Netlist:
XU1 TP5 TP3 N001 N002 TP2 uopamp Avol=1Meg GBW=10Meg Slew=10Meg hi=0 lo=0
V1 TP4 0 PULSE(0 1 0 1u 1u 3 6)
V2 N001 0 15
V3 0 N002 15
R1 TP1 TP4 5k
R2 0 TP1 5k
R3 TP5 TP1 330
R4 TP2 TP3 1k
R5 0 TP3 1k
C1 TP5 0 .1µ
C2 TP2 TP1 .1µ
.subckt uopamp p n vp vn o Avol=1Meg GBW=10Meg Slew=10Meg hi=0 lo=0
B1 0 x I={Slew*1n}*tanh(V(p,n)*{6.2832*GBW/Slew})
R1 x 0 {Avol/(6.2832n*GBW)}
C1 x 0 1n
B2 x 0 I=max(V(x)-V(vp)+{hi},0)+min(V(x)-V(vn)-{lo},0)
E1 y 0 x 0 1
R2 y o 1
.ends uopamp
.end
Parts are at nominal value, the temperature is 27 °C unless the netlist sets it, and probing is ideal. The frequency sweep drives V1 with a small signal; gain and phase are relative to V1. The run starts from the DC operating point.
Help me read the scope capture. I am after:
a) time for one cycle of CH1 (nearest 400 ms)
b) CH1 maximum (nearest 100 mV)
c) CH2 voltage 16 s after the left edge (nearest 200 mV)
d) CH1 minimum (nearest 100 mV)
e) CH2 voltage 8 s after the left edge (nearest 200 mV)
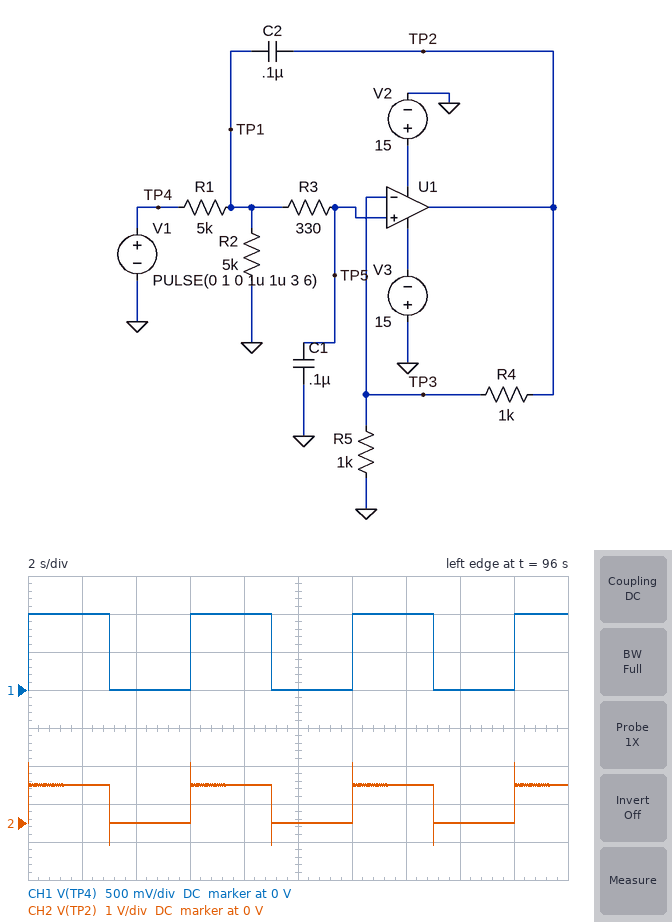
6.0 s
1.0 V
0 V
0 V
1.0 V
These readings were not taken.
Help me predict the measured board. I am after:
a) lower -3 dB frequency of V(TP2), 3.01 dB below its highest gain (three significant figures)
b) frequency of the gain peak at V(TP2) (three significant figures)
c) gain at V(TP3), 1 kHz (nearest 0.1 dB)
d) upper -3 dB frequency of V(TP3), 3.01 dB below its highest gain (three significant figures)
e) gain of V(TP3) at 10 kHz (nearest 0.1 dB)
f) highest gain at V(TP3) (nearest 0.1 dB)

1.33 kHz
1.69 kHz
-3.0 dB
1.99 kHz
-36.0 dB
2.9 dB
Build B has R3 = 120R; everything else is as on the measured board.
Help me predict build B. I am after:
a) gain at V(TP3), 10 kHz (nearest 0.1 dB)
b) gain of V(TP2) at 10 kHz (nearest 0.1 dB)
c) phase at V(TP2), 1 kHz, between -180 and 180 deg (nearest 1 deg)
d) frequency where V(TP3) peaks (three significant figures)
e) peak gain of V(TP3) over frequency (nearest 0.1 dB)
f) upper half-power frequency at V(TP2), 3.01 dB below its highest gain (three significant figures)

-26.8 dB
-20.8 dB
-5 deg
2.86 kHz
7.2 dB
3.17 kHz
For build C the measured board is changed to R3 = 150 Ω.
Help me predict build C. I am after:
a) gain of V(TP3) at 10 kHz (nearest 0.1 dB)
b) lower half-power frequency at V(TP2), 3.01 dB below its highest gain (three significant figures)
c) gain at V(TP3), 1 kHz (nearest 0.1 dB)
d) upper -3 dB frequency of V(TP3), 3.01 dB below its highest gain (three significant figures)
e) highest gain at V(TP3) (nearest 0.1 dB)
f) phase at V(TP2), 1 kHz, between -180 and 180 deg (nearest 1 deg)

-28.9 dB
2.21 kHz
-4.7 dB
2.86 kHz
6.3 dB
-6 deg
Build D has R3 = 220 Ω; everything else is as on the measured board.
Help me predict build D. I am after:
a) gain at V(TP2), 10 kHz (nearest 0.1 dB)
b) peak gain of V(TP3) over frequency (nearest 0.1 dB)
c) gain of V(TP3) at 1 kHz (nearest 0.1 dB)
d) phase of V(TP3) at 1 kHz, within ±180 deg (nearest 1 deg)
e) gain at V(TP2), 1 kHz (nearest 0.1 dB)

-26.4 dB
4.6 dB
-4.0 dB
-10 deg
2.0 dB
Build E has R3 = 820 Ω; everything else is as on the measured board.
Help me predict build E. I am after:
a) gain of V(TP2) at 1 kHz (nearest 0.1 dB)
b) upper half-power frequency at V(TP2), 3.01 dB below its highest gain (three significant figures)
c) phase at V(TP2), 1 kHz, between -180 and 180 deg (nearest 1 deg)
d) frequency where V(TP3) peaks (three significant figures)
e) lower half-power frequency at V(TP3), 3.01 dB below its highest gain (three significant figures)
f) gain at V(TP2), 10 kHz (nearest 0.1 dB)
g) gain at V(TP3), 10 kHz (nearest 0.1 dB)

5.2 dB
1.31 kHz
-70 deg
1.02 kHz
596 Hz
-38.1 dB
-44.1 dB
